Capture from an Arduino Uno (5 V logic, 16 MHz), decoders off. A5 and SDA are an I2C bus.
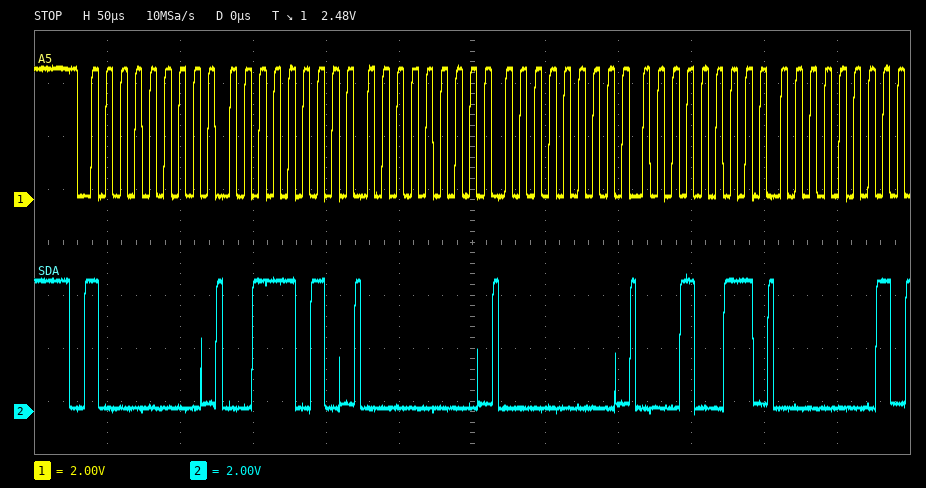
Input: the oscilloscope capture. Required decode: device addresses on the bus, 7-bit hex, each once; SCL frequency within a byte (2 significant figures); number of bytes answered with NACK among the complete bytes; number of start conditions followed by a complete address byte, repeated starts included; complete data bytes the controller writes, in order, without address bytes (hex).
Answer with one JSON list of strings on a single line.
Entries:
["0x40", "100 kHz", "0", "1", "3A 00 00 13 01"]
